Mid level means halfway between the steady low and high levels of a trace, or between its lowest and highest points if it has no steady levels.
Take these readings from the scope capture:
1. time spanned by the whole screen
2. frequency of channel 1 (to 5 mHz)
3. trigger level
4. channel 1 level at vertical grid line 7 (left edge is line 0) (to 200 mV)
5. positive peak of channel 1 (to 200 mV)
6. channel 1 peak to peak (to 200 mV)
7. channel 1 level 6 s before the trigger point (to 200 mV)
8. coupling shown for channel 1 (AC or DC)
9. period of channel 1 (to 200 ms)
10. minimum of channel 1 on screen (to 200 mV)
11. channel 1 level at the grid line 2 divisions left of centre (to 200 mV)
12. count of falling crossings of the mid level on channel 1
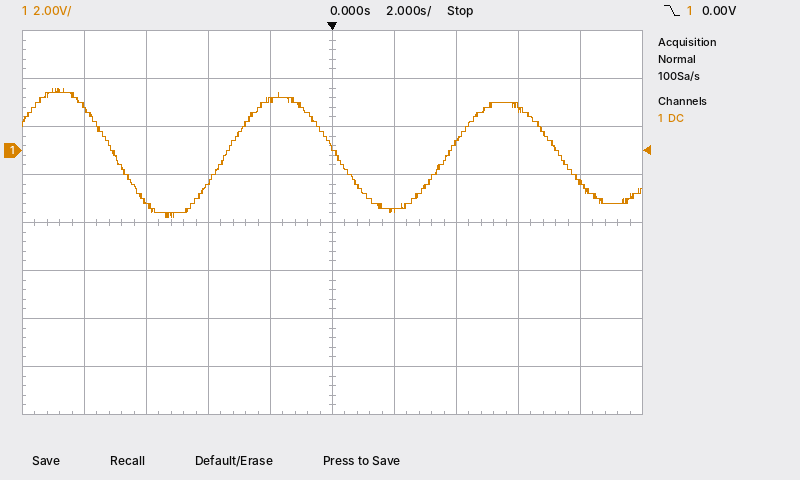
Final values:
20 s
140 mHz
0.00 V
400 mV
2.6 V
5.4 V
-2.2 V
DC
7.2 s
-2.8 V
-1.4 V
3
